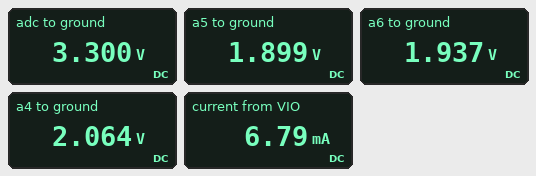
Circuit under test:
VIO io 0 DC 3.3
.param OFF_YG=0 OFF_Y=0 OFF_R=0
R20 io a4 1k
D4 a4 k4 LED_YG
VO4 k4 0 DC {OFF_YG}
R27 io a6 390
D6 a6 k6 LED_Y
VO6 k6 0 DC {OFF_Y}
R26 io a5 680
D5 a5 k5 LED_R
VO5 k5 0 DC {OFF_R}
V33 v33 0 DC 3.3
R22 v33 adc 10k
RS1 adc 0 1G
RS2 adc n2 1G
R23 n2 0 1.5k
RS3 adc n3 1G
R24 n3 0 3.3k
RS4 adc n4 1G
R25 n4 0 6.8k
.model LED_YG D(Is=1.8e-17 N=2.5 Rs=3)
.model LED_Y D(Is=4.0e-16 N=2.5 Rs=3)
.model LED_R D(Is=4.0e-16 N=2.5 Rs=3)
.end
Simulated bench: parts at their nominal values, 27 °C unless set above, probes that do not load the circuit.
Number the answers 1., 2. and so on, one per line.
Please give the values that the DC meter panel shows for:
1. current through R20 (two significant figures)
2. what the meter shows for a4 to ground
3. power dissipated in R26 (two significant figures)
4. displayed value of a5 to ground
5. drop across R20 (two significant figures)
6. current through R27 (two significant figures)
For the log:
1. 1.2 mA
2. 2.064 V
3. 2.9 mW
4. 1.899 V
5. 1.2 V
6. 3.5 mA
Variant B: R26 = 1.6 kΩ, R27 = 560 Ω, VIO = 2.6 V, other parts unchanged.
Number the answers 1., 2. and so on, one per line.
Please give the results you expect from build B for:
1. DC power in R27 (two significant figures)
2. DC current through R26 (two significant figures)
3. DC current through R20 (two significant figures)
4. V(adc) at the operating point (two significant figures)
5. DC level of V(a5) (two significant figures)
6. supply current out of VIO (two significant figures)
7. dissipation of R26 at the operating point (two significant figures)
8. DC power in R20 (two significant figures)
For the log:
1. 960 µW
2. 500 µA
3. 590 µA
4. 3.3 V
5. 1.8 V
6. 2.4 mA
7. 400 µW
8. 340 µW
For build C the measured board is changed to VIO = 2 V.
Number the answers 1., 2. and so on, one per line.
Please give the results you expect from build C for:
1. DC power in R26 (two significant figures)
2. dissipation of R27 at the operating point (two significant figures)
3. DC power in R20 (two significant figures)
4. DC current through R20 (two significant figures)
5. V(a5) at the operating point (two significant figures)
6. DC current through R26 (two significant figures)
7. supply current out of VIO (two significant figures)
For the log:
1. 74 µW
2. 99 µW
3. 10 µW
4. 100 µA
5. 1.8 V
6. 330 µA
7. 940 µA
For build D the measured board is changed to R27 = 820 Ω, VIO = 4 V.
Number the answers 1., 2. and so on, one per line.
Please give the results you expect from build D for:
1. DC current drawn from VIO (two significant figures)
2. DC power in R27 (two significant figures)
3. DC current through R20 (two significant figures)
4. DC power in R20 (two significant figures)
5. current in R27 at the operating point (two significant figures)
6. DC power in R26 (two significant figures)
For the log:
1. 7.5 mA
2. 5.3 mW
3. 1.9 mA
4. 3.6 mW
5. 2.5 mA
6. 6.3 mW
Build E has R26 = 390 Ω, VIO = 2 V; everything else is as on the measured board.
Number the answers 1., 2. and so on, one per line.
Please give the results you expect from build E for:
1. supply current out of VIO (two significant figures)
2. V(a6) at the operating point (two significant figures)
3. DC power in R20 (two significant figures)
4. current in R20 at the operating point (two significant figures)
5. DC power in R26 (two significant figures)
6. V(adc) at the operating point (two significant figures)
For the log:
1. 1.1 mA
2. 1.8 V
3. 10 µW
4. 100 µA
5. 99 µW
6. 3.3 V
